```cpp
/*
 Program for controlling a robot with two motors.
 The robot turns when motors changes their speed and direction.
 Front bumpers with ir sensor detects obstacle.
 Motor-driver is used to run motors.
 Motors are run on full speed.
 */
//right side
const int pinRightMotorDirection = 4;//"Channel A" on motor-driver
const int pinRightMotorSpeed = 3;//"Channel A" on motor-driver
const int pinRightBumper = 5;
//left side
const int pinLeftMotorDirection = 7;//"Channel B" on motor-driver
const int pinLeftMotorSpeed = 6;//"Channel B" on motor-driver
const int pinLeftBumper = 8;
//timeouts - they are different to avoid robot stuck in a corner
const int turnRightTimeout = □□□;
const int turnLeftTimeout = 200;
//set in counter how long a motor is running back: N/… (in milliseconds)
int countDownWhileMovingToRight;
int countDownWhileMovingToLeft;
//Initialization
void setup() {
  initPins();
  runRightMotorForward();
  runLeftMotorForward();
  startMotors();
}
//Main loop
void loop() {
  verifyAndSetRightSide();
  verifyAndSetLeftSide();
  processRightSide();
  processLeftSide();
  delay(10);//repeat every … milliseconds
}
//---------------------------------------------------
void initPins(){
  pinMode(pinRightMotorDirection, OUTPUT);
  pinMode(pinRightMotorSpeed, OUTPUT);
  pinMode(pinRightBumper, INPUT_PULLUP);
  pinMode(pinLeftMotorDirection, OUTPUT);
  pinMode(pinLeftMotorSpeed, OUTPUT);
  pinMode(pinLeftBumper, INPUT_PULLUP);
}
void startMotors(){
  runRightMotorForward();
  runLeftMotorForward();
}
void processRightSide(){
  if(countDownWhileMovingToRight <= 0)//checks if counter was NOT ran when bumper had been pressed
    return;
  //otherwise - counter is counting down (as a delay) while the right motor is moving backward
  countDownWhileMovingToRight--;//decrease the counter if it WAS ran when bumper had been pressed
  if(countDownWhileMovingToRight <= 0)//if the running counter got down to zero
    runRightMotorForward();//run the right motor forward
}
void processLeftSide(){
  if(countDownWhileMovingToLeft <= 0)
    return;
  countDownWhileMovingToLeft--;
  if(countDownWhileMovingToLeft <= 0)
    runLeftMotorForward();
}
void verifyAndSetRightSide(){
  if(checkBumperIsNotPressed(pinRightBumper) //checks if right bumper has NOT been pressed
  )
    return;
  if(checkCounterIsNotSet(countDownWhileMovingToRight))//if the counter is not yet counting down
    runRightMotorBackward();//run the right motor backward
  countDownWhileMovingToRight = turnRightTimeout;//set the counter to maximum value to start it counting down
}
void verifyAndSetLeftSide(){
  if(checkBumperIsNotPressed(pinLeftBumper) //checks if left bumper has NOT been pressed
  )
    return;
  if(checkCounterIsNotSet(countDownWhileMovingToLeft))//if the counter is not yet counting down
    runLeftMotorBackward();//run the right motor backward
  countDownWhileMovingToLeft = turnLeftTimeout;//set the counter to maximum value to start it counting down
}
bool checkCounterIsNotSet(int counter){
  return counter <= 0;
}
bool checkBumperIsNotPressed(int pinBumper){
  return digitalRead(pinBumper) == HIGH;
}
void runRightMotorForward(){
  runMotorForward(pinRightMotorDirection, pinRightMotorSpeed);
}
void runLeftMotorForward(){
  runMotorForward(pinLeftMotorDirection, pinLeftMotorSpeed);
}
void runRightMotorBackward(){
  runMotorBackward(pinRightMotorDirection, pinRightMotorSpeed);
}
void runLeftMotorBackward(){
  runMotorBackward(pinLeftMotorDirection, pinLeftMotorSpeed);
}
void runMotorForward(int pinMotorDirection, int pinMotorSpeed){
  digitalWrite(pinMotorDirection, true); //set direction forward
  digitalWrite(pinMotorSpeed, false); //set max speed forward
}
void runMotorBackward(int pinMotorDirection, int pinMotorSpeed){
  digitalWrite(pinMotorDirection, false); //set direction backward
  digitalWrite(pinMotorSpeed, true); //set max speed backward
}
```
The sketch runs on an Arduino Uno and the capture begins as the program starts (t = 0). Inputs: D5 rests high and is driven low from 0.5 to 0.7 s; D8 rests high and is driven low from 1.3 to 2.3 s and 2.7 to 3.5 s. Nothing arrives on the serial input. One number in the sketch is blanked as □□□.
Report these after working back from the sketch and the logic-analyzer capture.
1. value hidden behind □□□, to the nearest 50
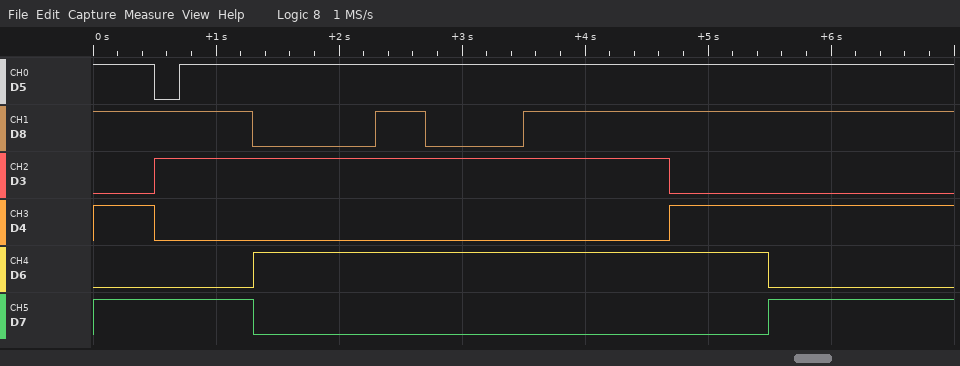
400
